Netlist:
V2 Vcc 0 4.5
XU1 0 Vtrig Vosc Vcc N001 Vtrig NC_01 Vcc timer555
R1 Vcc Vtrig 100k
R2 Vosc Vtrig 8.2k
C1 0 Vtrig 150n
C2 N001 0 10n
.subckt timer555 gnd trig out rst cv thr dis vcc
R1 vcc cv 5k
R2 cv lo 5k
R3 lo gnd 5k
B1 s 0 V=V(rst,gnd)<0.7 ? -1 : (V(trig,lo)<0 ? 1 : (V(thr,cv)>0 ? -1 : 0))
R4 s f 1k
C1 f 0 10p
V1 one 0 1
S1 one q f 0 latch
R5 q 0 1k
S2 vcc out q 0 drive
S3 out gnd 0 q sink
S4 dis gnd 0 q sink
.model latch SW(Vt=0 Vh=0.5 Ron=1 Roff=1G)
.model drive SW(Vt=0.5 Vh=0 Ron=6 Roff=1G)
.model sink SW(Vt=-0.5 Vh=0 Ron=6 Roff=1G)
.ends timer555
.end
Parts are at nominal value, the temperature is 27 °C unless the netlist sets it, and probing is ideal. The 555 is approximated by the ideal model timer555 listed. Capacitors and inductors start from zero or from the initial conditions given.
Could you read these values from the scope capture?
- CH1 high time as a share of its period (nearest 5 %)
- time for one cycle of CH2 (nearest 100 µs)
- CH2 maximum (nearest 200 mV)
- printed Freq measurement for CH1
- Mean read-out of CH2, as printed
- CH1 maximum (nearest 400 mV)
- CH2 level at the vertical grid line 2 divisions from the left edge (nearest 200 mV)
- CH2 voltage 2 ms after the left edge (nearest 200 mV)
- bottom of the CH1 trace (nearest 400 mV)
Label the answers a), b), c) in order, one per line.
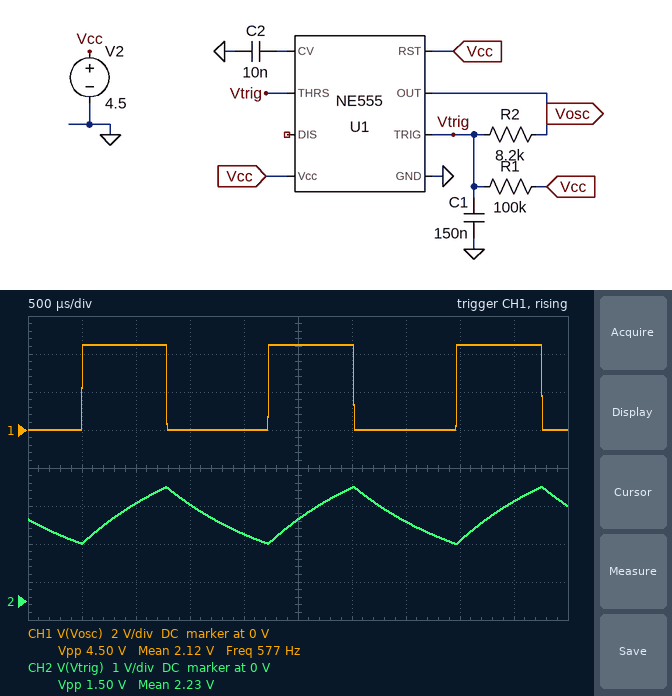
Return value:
a) 45 %
b) 1.7 ms
c) 3.0 V
d) 577 Hz
e) 2.23 V
f) 4.4 V
g) 2.6 V
h) 1.8 V
i) 0 V
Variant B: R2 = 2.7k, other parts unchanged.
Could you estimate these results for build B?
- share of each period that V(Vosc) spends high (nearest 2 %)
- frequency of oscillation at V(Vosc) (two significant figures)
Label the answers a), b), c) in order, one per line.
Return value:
a) 48 %
b) 1.8 kHz
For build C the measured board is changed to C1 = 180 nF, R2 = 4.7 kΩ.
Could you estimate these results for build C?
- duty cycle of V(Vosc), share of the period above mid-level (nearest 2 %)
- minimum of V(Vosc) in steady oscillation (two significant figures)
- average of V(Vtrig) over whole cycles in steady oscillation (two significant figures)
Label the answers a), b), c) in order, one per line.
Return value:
a) 48 %
b) 1.9 mV
c) 2.2 V
